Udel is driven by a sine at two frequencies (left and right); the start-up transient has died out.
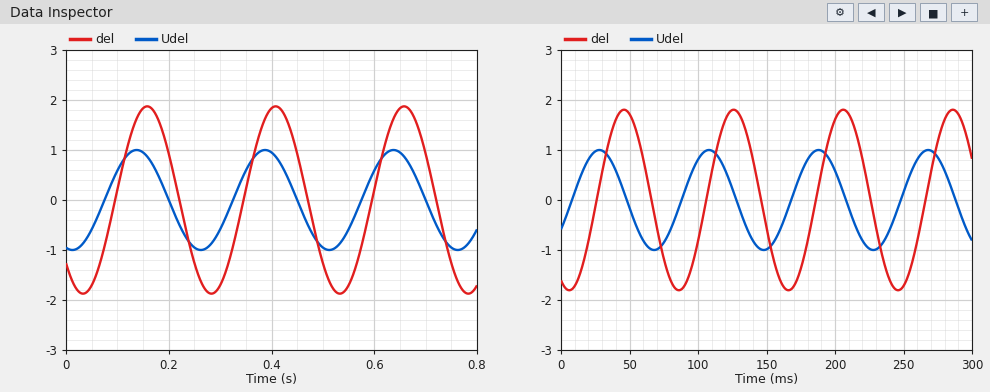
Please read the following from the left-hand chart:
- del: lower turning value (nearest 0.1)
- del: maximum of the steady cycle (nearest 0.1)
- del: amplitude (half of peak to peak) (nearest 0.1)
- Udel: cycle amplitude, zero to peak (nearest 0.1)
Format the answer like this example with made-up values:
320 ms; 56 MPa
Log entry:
-1.9; 1.9; 1.9; 1.0
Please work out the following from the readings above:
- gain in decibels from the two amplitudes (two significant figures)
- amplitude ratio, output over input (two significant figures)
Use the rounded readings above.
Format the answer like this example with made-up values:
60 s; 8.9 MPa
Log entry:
5.6 dB; 1.9
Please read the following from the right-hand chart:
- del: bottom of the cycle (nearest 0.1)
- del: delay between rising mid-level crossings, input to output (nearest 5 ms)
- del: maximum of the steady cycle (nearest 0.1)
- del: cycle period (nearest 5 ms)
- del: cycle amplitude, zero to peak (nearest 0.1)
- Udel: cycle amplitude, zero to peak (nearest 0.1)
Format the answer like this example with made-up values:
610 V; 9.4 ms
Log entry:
-1.8; 20 ms; 1.8; 80 ms; 1.8; 1.0
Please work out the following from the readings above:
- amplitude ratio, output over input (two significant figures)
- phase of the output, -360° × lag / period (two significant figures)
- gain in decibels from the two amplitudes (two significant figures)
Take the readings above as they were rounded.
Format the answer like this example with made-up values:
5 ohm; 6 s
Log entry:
1.8; -90°; 5.1 dB
